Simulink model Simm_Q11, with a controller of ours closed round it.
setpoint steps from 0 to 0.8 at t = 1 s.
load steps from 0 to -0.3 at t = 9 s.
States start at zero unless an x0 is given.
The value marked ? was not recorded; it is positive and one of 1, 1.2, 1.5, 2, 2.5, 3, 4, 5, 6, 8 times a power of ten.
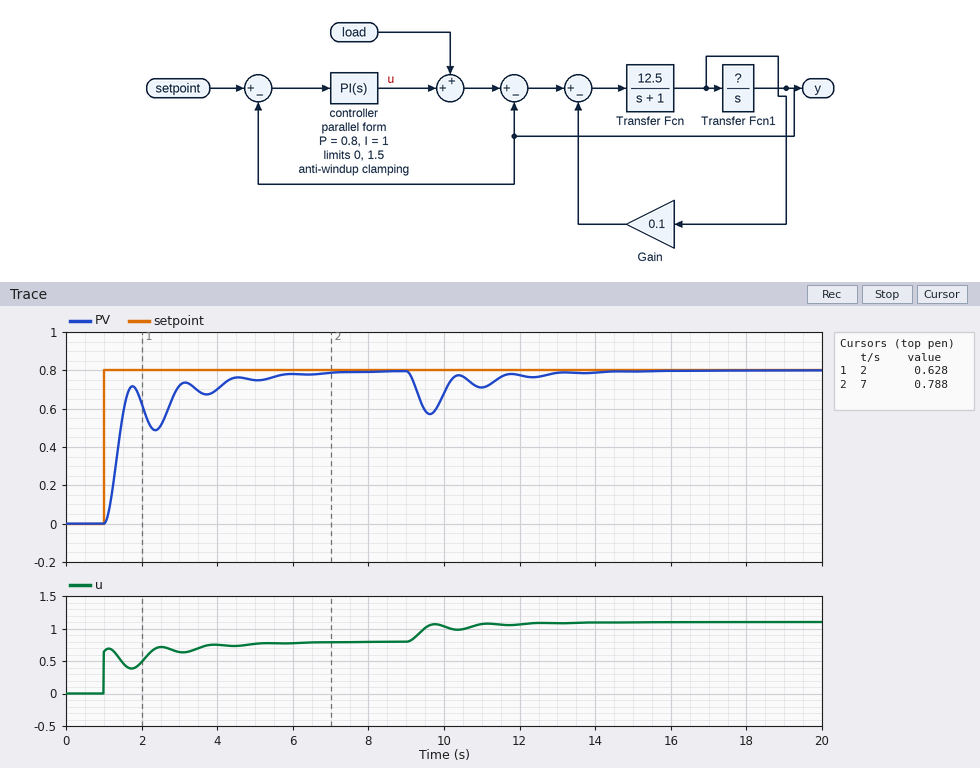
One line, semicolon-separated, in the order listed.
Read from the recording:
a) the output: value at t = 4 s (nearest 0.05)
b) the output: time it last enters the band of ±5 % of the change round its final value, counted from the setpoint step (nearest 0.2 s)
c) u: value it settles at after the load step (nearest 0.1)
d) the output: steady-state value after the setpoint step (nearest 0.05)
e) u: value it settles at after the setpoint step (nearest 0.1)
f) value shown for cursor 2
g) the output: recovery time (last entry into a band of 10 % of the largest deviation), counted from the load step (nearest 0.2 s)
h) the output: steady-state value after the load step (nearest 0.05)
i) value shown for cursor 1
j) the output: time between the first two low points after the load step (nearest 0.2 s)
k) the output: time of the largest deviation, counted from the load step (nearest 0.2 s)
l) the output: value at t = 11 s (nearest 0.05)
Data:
0.70; 4.4 s; 1.1; 0.80; 0.8; 0.788; 3.8 s; 0.80; 0.628; 1.4 s; 0.6 s; 0.70
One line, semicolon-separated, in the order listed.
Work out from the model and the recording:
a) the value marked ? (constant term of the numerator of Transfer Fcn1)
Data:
1
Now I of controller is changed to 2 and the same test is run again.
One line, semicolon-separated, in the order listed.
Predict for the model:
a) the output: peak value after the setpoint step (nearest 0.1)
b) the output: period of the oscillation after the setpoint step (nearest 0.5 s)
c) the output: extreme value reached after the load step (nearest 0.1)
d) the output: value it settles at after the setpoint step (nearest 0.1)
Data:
0.9; 1.5 s; 0.6; 0.8
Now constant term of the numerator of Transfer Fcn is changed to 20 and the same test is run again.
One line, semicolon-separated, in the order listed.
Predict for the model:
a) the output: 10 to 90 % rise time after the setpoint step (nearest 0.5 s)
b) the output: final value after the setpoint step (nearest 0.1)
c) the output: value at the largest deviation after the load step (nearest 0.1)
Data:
2.5 s; 0.8; 0.6
